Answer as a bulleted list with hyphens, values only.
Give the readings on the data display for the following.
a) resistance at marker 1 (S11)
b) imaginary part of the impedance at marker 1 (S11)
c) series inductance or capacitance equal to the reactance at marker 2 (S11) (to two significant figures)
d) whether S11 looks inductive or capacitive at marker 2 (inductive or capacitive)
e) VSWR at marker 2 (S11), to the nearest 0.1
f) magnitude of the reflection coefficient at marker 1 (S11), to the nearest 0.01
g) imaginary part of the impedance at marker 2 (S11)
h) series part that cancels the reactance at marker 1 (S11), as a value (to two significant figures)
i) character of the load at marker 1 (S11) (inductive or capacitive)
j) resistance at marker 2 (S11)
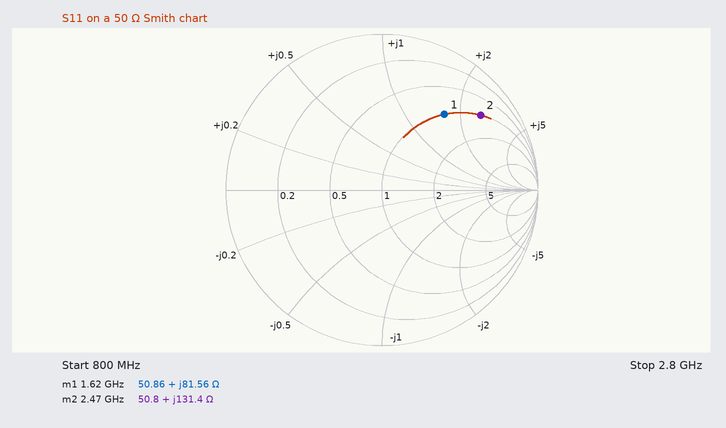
- 50.86 Ω
- +81.56 Ω
- 8.5 nH
- inductive
- 8.7
- 0.63
- +131.4 Ω
- 1.2 pF
- inductive
- 50.8 Ω
